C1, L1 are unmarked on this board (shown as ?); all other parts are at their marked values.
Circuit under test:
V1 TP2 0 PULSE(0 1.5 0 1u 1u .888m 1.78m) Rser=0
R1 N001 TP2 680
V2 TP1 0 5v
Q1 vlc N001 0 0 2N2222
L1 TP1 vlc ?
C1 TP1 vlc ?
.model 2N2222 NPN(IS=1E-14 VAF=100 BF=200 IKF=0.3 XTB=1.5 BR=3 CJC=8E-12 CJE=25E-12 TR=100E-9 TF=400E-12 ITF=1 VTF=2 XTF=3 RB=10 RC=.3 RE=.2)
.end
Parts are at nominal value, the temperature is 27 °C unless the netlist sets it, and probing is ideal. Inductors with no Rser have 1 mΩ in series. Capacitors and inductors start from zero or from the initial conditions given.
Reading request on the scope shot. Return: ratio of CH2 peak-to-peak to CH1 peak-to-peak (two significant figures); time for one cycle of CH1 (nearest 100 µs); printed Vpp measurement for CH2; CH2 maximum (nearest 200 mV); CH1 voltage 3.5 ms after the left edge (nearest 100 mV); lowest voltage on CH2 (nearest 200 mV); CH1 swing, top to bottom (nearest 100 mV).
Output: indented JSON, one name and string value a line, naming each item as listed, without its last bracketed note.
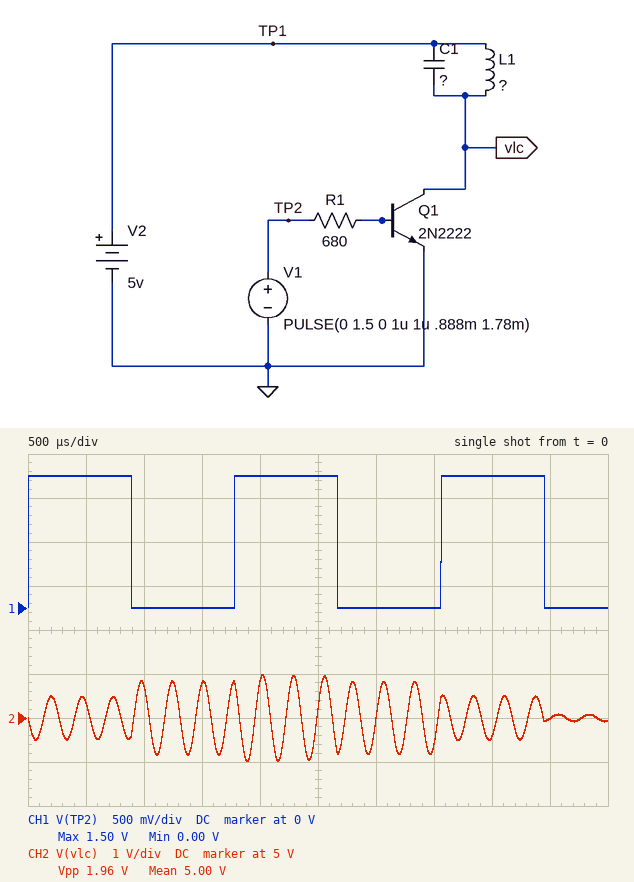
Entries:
{
  "ratio of CH2 peak-to-peak to CH1 peak-to-peak": "1.3",
  "time for one cycle of CH1": "1.8 ms",
  "printed Vpp measurement for CH2": "1.96 V",
  "CH2 maximum": "6.0 V",
  "CH1 voltage 3.5 ms after the left edge": "0 V",
  "lowest voltage on CH2": "4.0 V",
  "CH1 swing, top to bottom": "1.5 V"
}
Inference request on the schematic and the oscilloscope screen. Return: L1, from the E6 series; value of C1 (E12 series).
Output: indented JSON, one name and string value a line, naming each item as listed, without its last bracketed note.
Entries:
{
  "L1, from the E6 series": "150 µH",
  "value of C1": "12 µF"
}
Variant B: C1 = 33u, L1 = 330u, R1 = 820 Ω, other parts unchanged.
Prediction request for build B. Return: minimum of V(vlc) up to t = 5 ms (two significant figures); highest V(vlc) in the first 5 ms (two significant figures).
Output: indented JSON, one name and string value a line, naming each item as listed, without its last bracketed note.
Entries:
{
  "minimum of V(vlc) up to t = 5 ms": "4.1 V",
  "highest V(vlc) in the first 5 ms": "5.9 V"
}
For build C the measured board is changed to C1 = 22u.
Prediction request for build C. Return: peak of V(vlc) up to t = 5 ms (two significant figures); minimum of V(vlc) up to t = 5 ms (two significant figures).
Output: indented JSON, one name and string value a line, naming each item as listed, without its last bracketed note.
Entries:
{
  "peak of V(vlc) up to t = 5 ms": "7.0 V",
  "minimum of V(vlc) up to t = 5 ms": "3.0 V"
}
